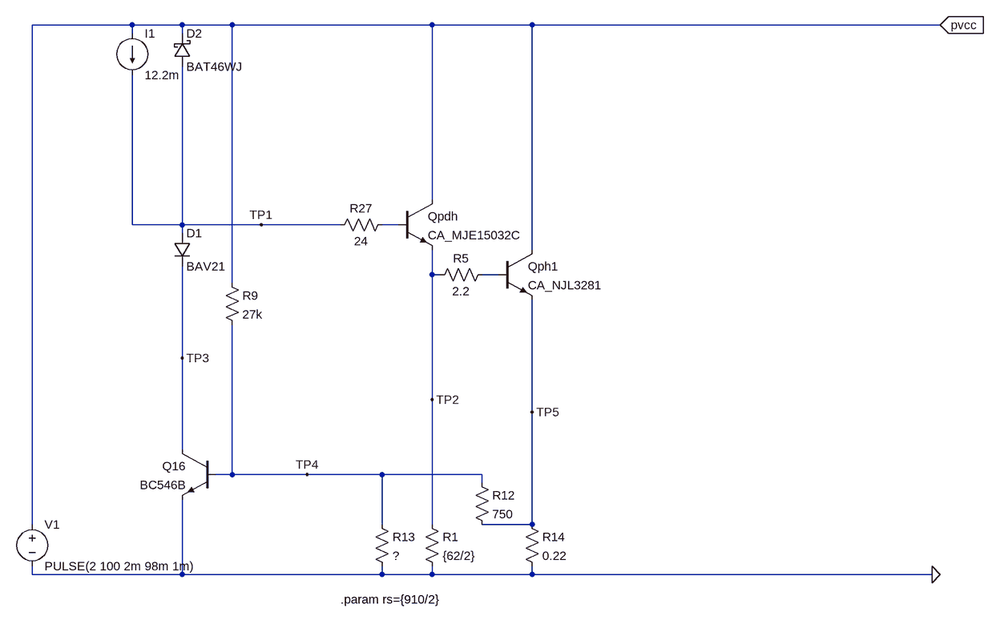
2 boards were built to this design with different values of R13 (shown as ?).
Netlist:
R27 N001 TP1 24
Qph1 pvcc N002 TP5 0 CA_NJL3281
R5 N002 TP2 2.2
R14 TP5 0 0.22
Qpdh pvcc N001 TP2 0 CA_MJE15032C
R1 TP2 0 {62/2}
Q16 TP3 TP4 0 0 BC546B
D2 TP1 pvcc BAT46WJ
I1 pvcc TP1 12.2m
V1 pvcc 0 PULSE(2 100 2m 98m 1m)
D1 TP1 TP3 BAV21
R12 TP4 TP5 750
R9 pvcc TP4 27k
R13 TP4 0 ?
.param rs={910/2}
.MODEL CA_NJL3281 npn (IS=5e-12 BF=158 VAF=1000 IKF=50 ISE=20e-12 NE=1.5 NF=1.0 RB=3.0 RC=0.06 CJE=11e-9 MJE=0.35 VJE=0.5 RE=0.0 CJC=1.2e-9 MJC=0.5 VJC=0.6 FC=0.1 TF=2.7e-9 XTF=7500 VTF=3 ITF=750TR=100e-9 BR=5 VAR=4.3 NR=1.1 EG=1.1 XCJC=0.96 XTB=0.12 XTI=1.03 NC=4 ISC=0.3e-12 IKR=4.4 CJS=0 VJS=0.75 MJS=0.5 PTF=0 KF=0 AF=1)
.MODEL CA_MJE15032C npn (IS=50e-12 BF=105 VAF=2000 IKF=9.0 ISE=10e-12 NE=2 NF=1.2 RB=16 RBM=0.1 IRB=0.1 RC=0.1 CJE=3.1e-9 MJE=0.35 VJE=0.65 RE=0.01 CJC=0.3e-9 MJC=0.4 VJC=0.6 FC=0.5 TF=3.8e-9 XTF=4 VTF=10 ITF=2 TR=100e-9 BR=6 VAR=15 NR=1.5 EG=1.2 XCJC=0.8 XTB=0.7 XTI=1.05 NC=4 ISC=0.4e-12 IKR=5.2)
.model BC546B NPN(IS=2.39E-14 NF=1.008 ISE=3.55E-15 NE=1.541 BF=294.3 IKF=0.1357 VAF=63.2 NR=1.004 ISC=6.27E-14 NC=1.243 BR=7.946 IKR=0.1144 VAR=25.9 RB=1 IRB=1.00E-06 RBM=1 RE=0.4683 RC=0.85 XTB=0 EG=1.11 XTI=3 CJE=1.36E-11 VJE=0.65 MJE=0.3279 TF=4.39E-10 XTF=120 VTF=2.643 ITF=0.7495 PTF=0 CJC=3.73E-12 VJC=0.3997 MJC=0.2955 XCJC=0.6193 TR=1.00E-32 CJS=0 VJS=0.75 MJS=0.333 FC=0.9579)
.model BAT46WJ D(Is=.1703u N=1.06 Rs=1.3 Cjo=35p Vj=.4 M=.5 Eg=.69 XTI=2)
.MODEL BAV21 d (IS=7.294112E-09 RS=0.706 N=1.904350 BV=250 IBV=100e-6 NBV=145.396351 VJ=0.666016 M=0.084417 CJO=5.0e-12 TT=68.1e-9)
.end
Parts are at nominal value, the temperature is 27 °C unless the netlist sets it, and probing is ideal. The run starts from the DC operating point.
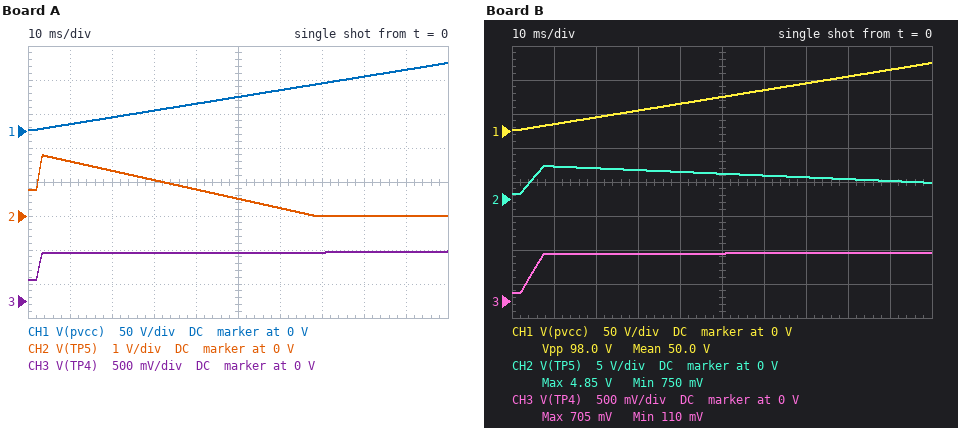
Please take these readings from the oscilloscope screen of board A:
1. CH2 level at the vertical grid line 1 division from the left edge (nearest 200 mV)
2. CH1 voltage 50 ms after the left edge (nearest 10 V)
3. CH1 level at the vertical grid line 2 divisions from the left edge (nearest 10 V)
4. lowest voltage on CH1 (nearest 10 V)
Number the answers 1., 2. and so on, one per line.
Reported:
1. 1.6 V
2. 50 V
3. 20 V
4. 0 V
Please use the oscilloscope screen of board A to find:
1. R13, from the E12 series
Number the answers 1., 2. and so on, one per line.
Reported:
1. 470 Ω
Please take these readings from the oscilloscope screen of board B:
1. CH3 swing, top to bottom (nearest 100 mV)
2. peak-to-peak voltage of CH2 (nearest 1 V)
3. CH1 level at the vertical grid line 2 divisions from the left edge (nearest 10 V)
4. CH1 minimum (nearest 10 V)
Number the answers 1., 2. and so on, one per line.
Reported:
1. 600 mV
2. 4 V
3. 20 V
4. 0 V
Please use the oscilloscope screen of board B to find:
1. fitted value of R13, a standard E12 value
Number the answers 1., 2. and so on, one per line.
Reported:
1. 120 Ω
